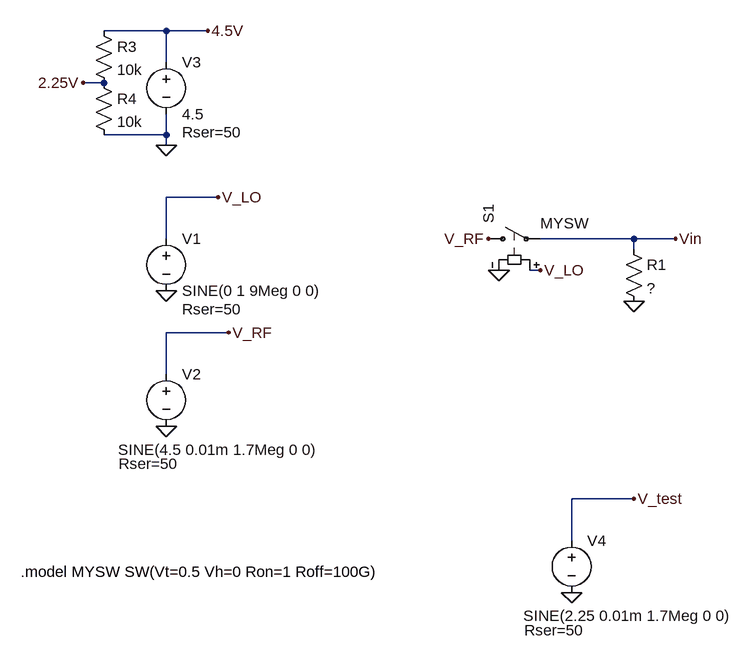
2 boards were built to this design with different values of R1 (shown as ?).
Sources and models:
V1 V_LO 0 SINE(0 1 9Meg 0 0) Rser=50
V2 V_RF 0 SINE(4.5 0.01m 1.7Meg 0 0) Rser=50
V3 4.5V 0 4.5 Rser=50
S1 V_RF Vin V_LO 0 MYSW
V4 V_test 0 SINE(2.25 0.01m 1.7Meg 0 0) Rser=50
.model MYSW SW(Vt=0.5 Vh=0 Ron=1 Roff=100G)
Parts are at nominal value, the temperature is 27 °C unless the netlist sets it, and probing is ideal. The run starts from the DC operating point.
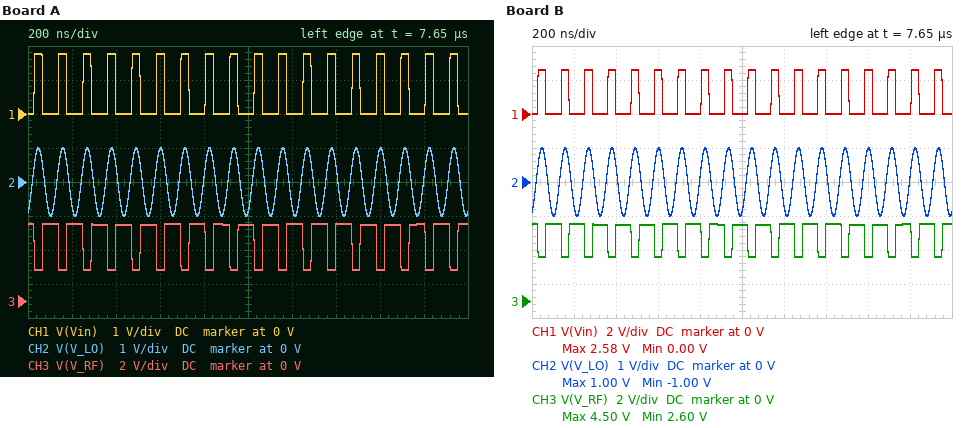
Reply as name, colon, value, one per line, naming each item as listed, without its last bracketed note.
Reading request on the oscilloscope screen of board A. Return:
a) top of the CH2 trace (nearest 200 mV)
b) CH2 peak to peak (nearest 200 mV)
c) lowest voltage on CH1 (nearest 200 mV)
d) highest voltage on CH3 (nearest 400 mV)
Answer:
top of the CH2 trace: 1.0 V
CH2 peak to peak: 2.0 V
lowest voltage on CH1: 0 V
highest voltage on CH3: 4.4 V
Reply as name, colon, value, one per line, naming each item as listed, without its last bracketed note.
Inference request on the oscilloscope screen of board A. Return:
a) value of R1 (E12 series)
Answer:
value of R1: 33 Ω
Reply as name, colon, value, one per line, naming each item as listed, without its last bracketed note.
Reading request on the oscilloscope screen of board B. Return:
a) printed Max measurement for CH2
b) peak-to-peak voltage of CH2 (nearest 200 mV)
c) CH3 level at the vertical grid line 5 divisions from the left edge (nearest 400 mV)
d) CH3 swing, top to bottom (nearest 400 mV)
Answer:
printed Max measurement for CH2: 1.00 V
peak-to-peak voltage of CH2: 2.0 V
CH3 level at the vertical grid line 5 divisions from the left edge: 4.4 V
CH3 swing, top to bottom: 2.0 V
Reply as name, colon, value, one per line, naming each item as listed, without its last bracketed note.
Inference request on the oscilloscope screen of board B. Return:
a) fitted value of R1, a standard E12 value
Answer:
fitted value of R1, a standard E12 value: 68 Ω
